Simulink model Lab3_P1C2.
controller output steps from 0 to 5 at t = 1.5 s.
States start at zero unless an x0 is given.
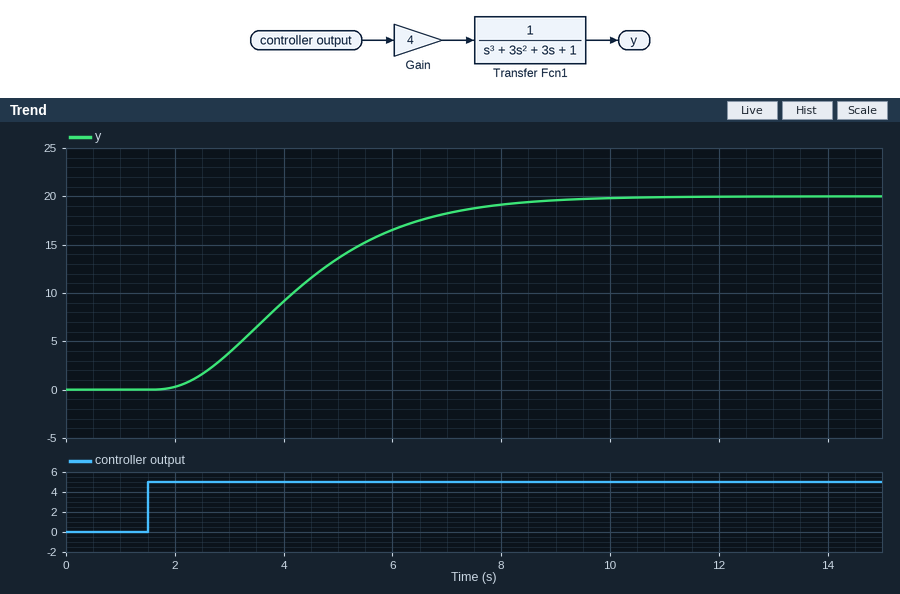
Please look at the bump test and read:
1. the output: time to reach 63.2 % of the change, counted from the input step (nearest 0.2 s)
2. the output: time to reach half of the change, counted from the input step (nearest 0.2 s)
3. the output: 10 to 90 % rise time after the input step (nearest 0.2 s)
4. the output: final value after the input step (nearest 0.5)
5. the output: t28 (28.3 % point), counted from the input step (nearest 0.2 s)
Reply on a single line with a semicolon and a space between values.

3.2 s; 2.6 s; 4.2 s; 20.0; 1.8 s
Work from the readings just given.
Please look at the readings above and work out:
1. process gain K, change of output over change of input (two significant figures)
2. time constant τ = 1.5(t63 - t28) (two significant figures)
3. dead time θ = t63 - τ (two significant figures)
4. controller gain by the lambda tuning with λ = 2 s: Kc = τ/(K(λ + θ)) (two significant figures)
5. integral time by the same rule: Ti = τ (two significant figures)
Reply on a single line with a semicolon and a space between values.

4.0; 2.1 s; 1.1 s; 0.17; 2.1 s
